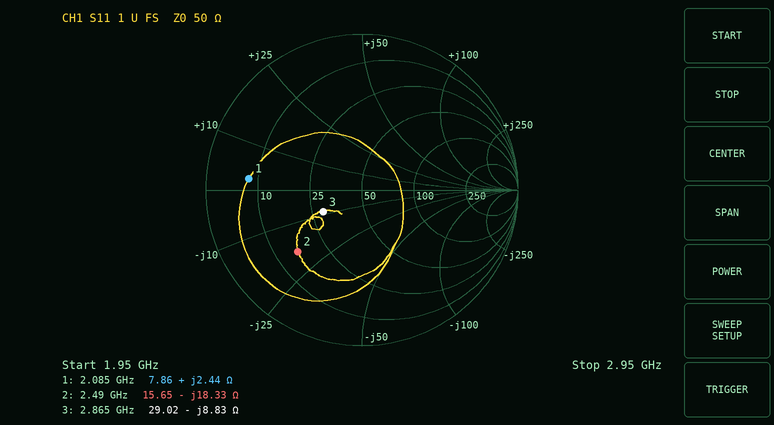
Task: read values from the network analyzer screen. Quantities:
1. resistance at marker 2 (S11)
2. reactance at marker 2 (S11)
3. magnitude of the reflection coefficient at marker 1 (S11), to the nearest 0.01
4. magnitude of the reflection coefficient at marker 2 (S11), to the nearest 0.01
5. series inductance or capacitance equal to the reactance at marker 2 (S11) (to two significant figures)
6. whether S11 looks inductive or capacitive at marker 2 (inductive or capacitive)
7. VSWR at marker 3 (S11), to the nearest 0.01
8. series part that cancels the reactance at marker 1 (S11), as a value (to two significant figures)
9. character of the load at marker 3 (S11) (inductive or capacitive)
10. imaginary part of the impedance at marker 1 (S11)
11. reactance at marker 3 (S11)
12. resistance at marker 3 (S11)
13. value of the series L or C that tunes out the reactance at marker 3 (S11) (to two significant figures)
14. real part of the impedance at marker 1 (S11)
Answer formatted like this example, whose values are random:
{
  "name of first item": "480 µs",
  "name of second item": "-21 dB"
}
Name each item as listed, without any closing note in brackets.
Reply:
{
  "resistance at marker 2": "15.65 Ω",
  "reactance at marker 2": "-18.33 Ω",
  "magnitude of the reflection coefficient at marker 1 (S11), to the nearest 0.01": "0.73",
  "magnitude of the reflection coefficient at marker 2 (S11), to the nearest 0.01": "0.57",
  "series inductance or capacitance equal to the reactance at marker 2 (S11)": "3.5 pF",
  "whether S11 looks inductive or capacitive at marker 2": "capacitive",
  "VSWR at marker 3 (S11), to the nearest 0.01": "1.80",
  "series part that cancels the reactance at marker 1 (S11), as a value": "31 pF",
  "character of the load at marker 3 (S11)": "capacitive",
  "imaginary part of the impedance at marker 1": "+2.44 Ω",
  "reactance at marker 3": "-8.83 Ω",
  "resistance at marker 3": "29.02 Ω",
  "value of the series L or C that tunes out the reactance at marker 3 (S11)": "490 pH",
  "real part of the impedance at marker 1": "7.86 Ω"
}
